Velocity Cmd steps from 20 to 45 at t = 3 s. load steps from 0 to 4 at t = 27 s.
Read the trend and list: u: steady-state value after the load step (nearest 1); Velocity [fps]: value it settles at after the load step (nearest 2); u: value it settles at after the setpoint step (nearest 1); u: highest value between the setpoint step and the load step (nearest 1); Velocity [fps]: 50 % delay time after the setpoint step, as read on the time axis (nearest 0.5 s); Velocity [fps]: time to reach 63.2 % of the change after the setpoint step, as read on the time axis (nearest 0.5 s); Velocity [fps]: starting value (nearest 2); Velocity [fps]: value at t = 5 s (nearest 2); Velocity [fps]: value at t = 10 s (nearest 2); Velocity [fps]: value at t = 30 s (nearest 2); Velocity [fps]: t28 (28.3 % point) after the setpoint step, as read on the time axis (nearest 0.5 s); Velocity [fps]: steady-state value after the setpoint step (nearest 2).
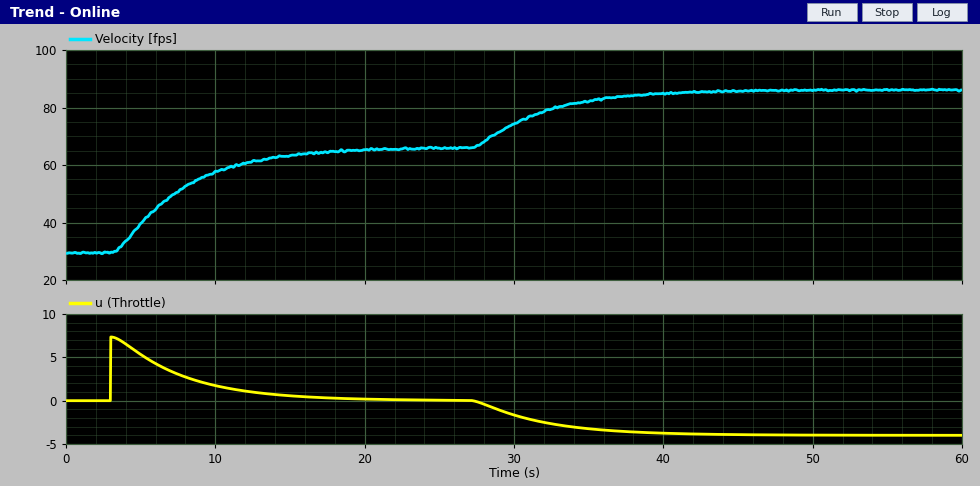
-4
86
0
7
6.5 s
8.0 s
30
40
58
74
5.0 s
66
